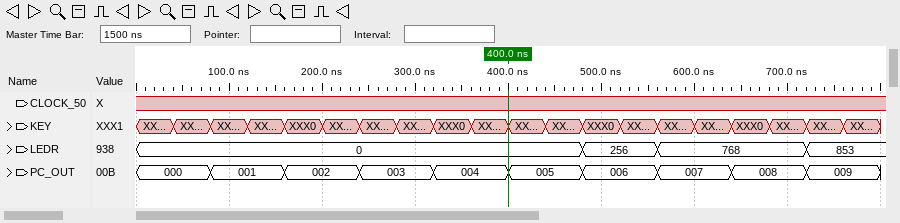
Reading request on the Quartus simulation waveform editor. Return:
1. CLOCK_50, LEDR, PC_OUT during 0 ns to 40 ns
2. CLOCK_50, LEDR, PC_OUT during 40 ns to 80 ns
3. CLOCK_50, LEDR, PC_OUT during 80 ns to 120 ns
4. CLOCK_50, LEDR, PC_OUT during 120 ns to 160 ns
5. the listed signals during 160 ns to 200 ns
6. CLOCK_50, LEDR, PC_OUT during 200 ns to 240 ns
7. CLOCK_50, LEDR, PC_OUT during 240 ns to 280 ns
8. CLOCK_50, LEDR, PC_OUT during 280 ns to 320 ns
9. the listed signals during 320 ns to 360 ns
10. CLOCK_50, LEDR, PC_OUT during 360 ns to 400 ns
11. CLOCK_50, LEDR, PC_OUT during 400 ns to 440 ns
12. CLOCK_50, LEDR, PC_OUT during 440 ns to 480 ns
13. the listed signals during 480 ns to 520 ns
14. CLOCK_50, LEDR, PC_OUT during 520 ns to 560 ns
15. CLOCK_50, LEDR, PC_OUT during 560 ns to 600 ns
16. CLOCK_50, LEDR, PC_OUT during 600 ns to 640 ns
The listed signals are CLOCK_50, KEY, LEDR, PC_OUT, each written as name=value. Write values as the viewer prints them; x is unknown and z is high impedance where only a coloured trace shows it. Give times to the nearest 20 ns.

CLOCK_50=x, LEDR=0, PC_OUT=000
CLOCK_50=x, LEDR=0, PC_OUT=000
CLOCK_50=x, LEDR=0, PC_OUT=001
CLOCK_50=x, LEDR=0, PC_OUT=001
CLOCK_50=x, KEY=XXX0, LEDR=0, PC_OUT=002
CLOCK_50=x, LEDR=0, PC_OUT=002
CLOCK_50=x, LEDR=0, PC_OUT=003
CLOCK_50=x, LEDR=0, PC_OUT=003
CLOCK_50=x, KEY=XXX0, LEDR=0, PC_OUT=004
CLOCK_50=x, LEDR=0, PC_OUT=004
CLOCK_50=x, LEDR=0, PC_OUT=005
CLOCK_50=x, LEDR=0, PC_OUT=005
CLOCK_50=x, KEY=XXX0, LEDR=256, PC_OUT=006
CLOCK_50=x, LEDR=256, PC_OUT=006
CLOCK_50=x, LEDR=768, PC_OUT=007
CLOCK_50=x, LEDR=768, PC_OUT=007
